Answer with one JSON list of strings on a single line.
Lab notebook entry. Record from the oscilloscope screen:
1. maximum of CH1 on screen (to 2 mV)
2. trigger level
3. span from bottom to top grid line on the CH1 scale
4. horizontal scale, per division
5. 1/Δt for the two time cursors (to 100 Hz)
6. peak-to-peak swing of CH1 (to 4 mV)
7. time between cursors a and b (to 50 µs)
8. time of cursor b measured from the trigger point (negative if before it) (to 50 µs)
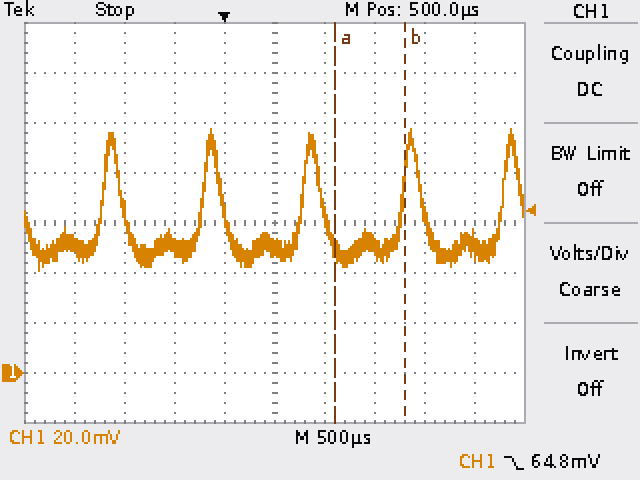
["98 mV", "64.8 mV", "160 mV", "500 µs", "1.4 kHz", "56 mV", "700 µs", "+1.80 ms"]
